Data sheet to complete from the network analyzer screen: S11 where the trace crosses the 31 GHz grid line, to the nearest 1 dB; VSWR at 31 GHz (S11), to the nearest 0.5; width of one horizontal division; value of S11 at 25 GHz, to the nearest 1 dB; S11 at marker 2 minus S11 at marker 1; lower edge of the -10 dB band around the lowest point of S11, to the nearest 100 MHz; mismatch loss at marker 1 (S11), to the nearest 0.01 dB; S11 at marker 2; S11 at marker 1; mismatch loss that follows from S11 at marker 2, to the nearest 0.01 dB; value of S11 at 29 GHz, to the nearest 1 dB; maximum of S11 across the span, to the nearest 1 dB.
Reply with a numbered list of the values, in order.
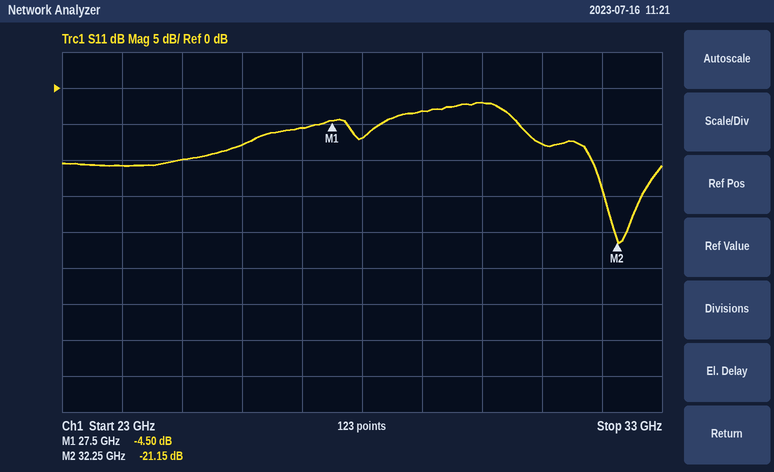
1. -8 dB
2. 2.5
3. 1 GHz
4. -10 dB
5. -16.65 dB
6. 31.8 GHz
7. 1.90 dB
8. -21.15 dB
9. -4.50 dB
10. 0.03 dB
11. -3 dB
12. -2 dB
